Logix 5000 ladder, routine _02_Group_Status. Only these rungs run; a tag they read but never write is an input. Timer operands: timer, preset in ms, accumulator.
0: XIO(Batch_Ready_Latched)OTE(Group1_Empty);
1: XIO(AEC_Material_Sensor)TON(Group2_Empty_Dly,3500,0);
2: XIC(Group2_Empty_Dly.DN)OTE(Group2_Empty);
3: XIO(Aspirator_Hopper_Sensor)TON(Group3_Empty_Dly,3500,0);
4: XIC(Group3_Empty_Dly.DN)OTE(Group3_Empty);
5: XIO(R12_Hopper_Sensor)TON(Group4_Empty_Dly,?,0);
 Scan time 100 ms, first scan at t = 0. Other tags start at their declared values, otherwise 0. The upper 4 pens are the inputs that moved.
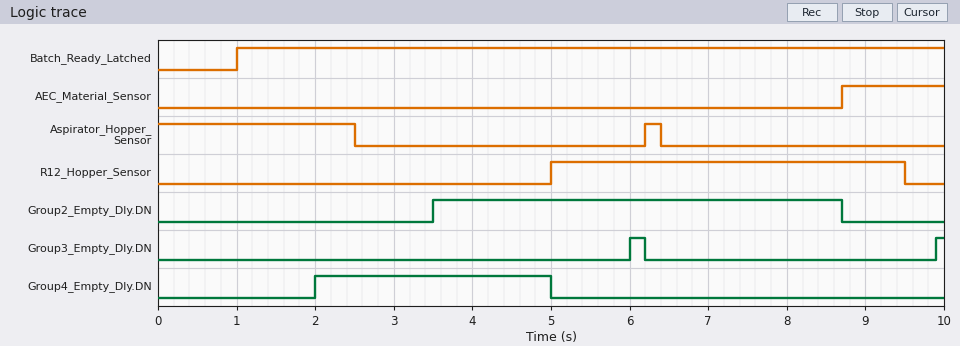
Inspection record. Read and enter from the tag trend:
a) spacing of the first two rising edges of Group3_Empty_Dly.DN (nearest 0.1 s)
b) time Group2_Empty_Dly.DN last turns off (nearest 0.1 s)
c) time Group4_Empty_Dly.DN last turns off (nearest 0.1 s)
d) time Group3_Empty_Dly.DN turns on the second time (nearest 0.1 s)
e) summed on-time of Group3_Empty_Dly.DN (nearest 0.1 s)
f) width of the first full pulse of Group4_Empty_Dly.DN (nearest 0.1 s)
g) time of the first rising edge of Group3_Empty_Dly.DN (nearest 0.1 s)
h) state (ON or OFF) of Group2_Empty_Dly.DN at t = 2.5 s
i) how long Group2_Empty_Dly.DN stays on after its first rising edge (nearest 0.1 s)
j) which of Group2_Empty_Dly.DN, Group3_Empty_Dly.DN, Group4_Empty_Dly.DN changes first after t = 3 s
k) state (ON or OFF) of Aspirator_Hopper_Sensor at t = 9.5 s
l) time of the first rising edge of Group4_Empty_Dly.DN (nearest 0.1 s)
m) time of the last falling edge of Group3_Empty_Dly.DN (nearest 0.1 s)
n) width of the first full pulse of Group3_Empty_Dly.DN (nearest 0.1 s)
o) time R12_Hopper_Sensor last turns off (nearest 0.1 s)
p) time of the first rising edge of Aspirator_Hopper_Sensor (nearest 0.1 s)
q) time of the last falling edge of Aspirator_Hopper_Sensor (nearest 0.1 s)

3.9 s
8.7 s
5.0 s
9.9 s
0.3 s
3.0 s
6.0 s
OFF
5.2 s
Group2_Empty_Dly.DN
OFF
2.0 s
6.2 s
0.2 s
9.5 s
6.2 s
6.4 s
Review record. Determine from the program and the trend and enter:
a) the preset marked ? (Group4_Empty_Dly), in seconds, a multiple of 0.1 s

2.0 s
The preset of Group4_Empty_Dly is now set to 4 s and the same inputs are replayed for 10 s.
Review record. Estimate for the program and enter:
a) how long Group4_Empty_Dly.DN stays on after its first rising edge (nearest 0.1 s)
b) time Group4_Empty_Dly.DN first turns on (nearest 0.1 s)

1.0 s
4.0 s
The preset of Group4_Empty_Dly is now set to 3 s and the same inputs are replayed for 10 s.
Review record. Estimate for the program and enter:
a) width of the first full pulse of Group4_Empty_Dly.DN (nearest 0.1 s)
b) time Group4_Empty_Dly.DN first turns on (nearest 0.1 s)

2.0 s
3.0 s
